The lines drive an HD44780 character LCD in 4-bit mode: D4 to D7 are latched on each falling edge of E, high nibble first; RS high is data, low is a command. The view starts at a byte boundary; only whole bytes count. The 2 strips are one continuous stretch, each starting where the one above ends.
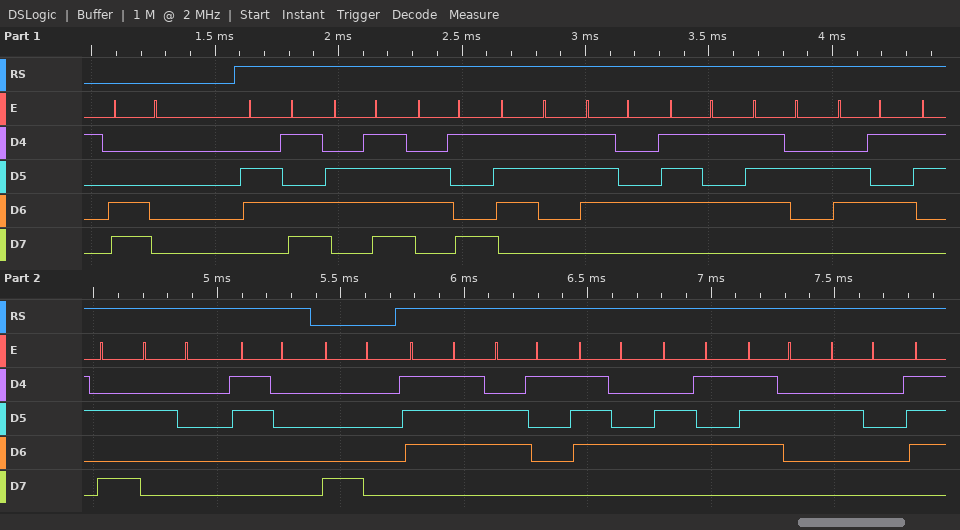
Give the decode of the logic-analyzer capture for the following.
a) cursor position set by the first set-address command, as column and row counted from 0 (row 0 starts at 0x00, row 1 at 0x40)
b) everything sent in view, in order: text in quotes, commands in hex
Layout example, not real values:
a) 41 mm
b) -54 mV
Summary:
a) column 0, row 1
b) 0xC0 "moisture: 0" 0x80 "water "
